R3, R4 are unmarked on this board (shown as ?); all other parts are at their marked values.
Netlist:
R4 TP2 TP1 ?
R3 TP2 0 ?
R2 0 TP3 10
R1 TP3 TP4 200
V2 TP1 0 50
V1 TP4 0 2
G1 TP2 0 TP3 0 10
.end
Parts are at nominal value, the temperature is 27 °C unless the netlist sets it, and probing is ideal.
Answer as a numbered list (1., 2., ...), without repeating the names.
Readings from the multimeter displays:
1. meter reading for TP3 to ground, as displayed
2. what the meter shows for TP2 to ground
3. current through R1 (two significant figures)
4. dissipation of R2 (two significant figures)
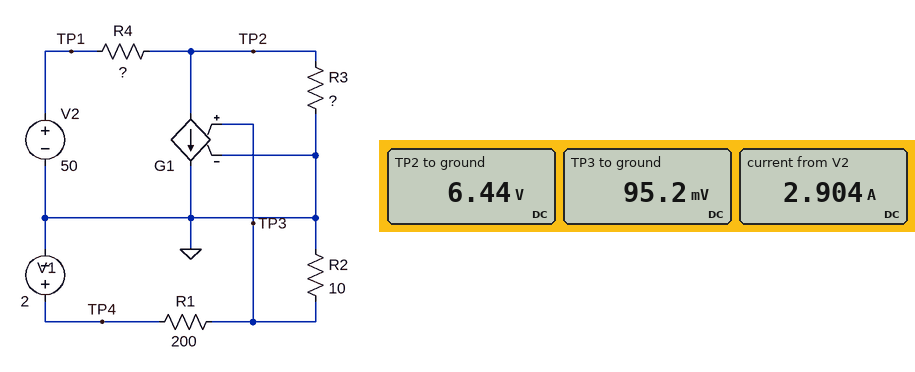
1. 95.2 mV
2. 6.44 V
3. 9.5 mA
4. 910 µW
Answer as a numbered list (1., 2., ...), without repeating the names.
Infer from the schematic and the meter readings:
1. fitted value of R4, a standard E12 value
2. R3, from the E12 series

1. 15 Ω
2. 3.3 Ω
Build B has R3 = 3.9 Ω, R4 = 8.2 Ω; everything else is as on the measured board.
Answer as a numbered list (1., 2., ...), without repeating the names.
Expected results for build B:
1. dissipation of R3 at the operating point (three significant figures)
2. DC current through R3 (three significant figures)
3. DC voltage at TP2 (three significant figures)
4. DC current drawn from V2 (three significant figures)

1. 47.4 W
2. 3.49 A
3. 13.6 V
4. 4.44 A
